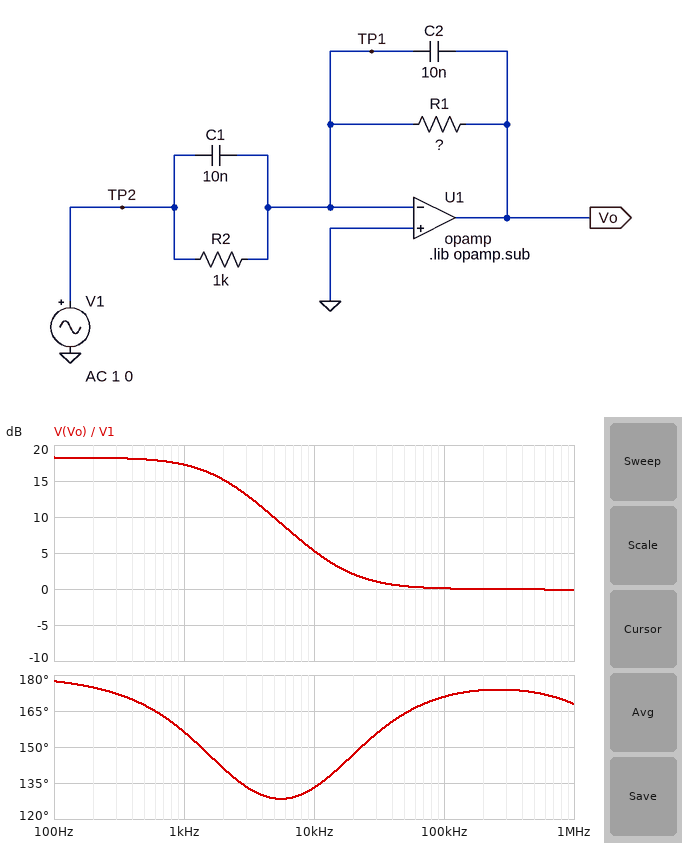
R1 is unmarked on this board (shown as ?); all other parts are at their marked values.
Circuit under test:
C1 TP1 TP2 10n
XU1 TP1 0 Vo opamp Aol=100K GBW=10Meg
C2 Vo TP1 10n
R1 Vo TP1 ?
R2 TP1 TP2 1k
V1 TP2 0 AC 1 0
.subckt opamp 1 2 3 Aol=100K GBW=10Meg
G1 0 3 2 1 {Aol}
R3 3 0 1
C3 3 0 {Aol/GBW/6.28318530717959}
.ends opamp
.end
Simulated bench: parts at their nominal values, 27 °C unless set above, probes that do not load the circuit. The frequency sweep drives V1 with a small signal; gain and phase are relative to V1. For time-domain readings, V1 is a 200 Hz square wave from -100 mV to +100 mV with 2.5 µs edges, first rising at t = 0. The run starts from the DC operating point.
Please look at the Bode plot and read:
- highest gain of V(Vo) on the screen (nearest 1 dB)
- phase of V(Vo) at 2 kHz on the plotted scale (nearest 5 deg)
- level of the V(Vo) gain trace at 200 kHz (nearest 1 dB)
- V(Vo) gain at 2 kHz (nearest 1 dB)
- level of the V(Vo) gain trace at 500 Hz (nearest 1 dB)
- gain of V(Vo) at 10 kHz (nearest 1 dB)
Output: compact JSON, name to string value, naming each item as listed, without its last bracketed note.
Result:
{"highest gain of V(Vo) on the screen": "18 dB", "phase of V(Vo) at 2 kHz on the plotted scale": "140 deg", "level of the V(Vo) gain trace at 200 kHz": "0 dB", "V(Vo) gain at 2 kHz": "15 dB", "level of the V(Vo) gain trace at 500 Hz": "18 dB", "gain of V(Vo) at 10 kHz": "5 dB"}
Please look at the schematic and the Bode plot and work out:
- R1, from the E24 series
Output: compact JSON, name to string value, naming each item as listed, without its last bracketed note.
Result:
{"R1, from the E24 series": "8.2 kΩ"}
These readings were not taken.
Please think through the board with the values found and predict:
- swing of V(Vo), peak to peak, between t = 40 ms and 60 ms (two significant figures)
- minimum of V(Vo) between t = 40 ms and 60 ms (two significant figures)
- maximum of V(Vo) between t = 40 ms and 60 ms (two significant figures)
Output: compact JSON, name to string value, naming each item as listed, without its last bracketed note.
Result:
{"swing of V(Vo), peak to peak, between t = 40 ms and 60 ms": "1.6 V", "minimum of V(Vo) between t = 40 ms and 60 ms": "-820 mV", "maximum of V(Vo) between t = 40 ms and 60 ms": "820 mV"}
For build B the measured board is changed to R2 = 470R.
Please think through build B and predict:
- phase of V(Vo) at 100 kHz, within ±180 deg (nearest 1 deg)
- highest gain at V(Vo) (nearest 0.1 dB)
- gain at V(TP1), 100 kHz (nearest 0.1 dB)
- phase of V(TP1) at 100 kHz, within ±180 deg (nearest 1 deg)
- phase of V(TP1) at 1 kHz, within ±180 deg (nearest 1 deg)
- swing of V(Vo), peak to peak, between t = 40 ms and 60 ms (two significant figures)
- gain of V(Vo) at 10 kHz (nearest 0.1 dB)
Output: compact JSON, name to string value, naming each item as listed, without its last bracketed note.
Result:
{"phase of V(Vo) at 100 kHz, within ±180 deg": "161 deg", "highest gain at V(Vo)": "24.8 dB", "gain at V(TP1), 100 kHz": "-39.6 dB", "phase of V(TP1) at 100 kHz, within ±180 deg": "71 deg", "phase of V(TP1) at 1 kHz, within ±180 deg": "59 deg", "swing of V(Vo), peak to peak, between t = 40 ms and 60 ms": "3.5 V", "gain of V(Vo) at 10 kHz": "10.8 dB"}
